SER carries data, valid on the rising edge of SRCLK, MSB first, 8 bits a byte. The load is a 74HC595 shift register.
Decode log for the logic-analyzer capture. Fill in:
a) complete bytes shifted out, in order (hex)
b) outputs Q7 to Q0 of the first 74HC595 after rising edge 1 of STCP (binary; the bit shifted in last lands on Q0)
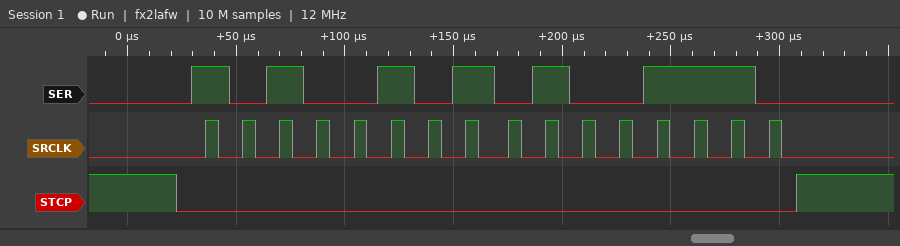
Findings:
A5 4E
01001110
